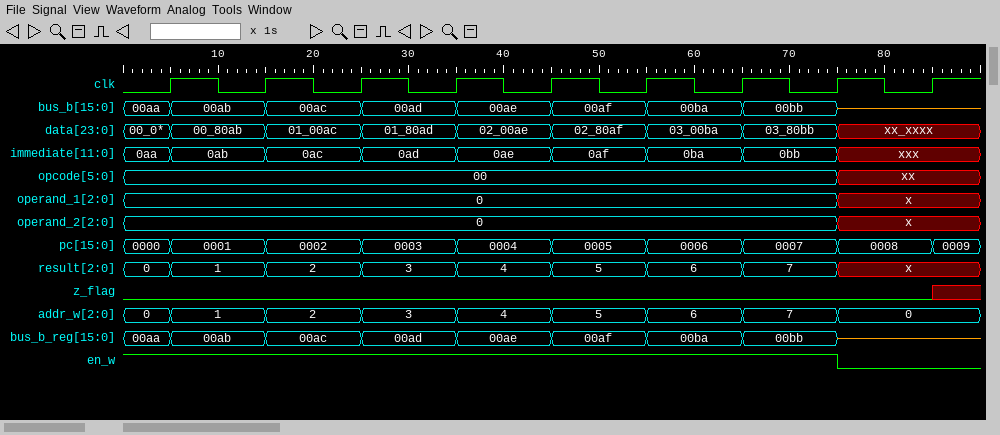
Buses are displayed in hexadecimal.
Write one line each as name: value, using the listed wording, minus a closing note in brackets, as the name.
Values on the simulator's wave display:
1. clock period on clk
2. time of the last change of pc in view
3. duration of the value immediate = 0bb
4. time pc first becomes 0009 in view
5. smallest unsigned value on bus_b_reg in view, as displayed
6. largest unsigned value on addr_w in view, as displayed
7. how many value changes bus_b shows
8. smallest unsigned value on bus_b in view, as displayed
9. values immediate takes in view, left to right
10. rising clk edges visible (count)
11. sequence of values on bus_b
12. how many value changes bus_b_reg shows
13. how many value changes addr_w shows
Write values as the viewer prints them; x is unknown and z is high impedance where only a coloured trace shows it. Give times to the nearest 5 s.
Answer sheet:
clock period on clk: 10 s
time of the last change of pc in view: 85 s
duration of the value immediate = 0bb: 10 s
time pc first becomes 0009 in view: 85 s
smallest unsigned value on bus_b_reg in view, as displayed: 00aa
largest unsigned value on addr_w in view, as displayed: 7
how many value changes bus_b shows: 8
smallest unsigned value on bus_b in view, as displayed: 00aa
values immediate takes in view, left to right: 0aa, 0ab, 0ac, 0ad, 0ae, 0af, 0ba, 0bb, xxx
rising clk edges visible: 9
sequence of values on bus_b: 00aa, 00ab, 00ac, 00ad, 00ae, 00af, 00ba, 00bb, z
how many value changes bus_b_reg shows: 8
how many value changes addr_w shows: 8
